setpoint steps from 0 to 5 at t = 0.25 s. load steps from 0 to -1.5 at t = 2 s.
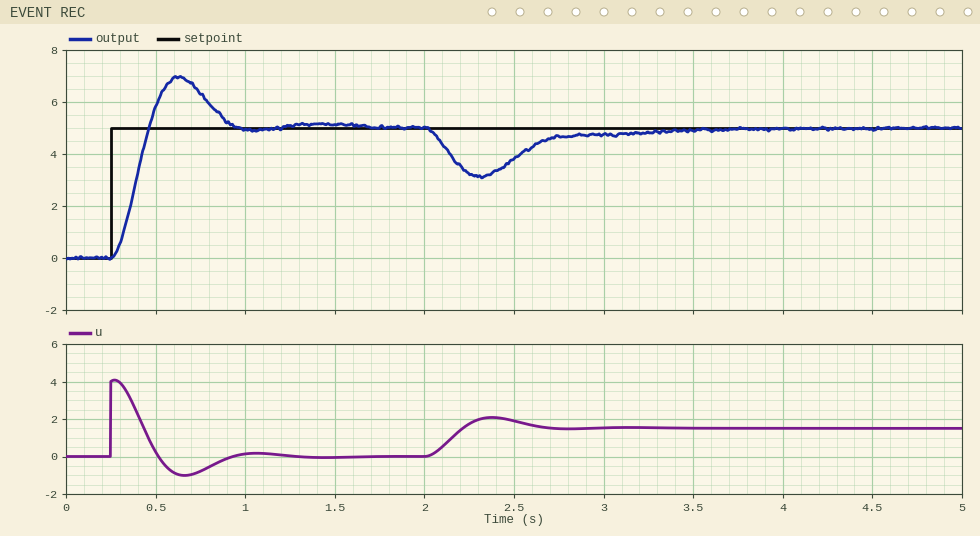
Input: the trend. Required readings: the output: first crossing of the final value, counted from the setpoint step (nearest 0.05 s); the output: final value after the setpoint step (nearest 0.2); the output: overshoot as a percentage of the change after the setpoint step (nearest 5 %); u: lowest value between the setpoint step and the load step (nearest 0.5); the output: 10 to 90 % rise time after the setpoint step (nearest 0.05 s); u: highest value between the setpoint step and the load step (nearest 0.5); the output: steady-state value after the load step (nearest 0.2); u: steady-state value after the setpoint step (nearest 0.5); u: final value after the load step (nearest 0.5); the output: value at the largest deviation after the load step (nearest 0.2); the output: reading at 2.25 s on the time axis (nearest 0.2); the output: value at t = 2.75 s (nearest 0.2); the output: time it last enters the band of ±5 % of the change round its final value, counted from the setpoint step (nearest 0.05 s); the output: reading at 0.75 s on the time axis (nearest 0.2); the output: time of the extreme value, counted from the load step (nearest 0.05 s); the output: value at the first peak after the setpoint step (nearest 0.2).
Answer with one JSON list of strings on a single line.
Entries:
["0.20 s", "5.0", "40 %", "-1.0", "0.15 s", "4.0", "5.0", "0.0", "1.5", "3.2", "3.2", "4.6", "0.65 s", "6.4", "0.30 s", "7.0"]
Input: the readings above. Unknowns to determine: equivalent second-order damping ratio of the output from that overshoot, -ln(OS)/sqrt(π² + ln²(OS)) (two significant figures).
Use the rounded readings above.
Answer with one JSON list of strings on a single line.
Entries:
["0.28"]
